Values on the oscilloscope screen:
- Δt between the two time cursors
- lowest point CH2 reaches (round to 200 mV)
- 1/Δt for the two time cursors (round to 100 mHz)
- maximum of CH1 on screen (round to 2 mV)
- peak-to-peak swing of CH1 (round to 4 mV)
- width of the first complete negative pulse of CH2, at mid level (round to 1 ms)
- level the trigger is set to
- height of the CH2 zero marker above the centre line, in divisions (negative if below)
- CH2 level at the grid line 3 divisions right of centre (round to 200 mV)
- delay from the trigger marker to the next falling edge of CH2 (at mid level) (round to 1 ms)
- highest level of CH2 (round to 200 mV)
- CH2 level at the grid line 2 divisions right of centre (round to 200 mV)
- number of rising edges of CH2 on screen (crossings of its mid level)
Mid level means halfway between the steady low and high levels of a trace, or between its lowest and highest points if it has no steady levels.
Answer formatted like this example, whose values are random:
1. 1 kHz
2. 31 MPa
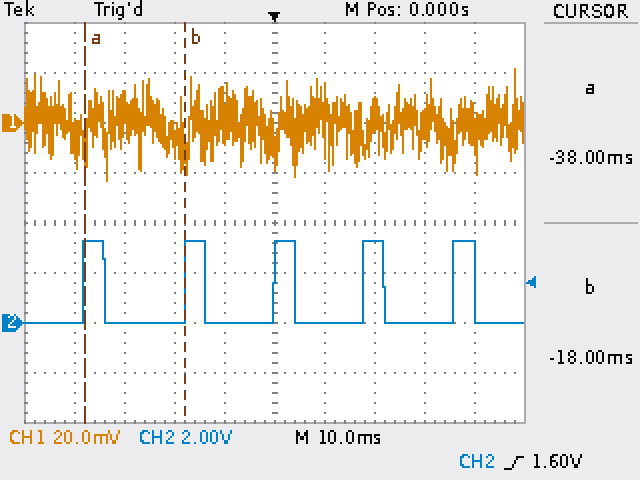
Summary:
1. 20 ms
2. 0.0 V
3. 50.0 Hz
4. 22 mV
5. 44 mV
6. 16 ms
7. 1.60 V
8. -2.0 div
9. 0.0 V
10. 4 ms
11. 3.2 V
12. 3.2 V
13. 5
